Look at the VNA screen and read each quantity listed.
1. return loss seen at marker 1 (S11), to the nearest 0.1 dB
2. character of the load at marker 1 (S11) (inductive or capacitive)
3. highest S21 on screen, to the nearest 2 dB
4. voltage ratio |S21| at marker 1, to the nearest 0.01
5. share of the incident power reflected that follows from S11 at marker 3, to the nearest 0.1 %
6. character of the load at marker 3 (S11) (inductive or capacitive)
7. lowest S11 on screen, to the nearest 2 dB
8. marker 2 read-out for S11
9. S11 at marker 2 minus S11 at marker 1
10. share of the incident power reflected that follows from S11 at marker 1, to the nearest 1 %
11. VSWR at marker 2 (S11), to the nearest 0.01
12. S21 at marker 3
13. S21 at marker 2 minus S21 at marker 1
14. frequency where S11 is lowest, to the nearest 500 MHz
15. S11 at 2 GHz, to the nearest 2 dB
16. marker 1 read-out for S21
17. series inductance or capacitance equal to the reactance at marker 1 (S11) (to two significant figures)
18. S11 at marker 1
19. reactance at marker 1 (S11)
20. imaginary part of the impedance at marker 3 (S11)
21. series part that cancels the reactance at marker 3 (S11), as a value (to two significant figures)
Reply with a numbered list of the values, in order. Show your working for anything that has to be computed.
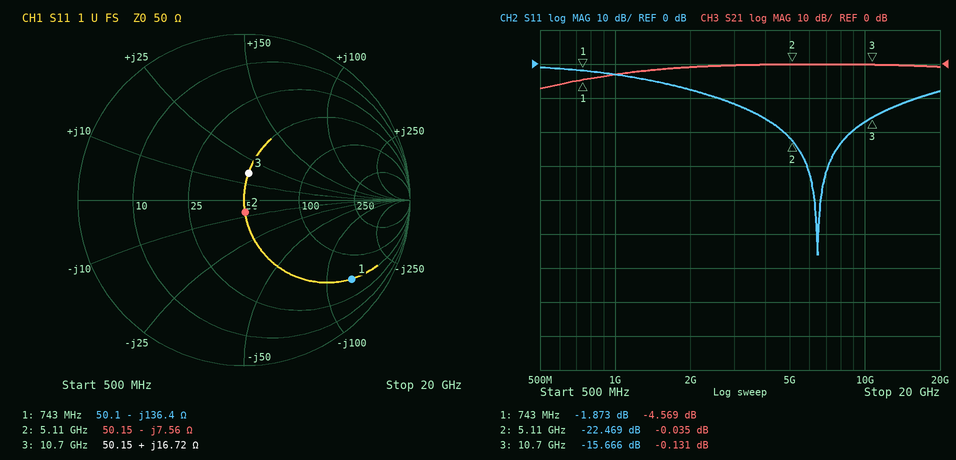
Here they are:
1. 1.9 dB
2. capacitive
3. 0 dB
4. 10^(-4.569/20) ≈ 0.59
5. 10^(-15.666/10) ≈ 2.7 %
6. inductive
7. -56 dB
8. -22.469 dB
9. -22.469 − (-1.873) = -20.596 dB
10. 10^(-1.873/10) ≈ 65 %
11. 1.16
12. -0.131 dB
13. -0.035 − (-4.569) = 4.534 dB
14. 6.5 GHz
15. -8 dB
16. -4.569 dB
17. C = 1/(2π × 743 MHz × 136.4 Ω) ≈ 1.6 pF
18. -1.873 dB
19. -136.4 Ω
20. +16.72 Ω
21. C = 1/(2π × 10.7 GHz × 16.72 Ω) ≈ 890 fF
